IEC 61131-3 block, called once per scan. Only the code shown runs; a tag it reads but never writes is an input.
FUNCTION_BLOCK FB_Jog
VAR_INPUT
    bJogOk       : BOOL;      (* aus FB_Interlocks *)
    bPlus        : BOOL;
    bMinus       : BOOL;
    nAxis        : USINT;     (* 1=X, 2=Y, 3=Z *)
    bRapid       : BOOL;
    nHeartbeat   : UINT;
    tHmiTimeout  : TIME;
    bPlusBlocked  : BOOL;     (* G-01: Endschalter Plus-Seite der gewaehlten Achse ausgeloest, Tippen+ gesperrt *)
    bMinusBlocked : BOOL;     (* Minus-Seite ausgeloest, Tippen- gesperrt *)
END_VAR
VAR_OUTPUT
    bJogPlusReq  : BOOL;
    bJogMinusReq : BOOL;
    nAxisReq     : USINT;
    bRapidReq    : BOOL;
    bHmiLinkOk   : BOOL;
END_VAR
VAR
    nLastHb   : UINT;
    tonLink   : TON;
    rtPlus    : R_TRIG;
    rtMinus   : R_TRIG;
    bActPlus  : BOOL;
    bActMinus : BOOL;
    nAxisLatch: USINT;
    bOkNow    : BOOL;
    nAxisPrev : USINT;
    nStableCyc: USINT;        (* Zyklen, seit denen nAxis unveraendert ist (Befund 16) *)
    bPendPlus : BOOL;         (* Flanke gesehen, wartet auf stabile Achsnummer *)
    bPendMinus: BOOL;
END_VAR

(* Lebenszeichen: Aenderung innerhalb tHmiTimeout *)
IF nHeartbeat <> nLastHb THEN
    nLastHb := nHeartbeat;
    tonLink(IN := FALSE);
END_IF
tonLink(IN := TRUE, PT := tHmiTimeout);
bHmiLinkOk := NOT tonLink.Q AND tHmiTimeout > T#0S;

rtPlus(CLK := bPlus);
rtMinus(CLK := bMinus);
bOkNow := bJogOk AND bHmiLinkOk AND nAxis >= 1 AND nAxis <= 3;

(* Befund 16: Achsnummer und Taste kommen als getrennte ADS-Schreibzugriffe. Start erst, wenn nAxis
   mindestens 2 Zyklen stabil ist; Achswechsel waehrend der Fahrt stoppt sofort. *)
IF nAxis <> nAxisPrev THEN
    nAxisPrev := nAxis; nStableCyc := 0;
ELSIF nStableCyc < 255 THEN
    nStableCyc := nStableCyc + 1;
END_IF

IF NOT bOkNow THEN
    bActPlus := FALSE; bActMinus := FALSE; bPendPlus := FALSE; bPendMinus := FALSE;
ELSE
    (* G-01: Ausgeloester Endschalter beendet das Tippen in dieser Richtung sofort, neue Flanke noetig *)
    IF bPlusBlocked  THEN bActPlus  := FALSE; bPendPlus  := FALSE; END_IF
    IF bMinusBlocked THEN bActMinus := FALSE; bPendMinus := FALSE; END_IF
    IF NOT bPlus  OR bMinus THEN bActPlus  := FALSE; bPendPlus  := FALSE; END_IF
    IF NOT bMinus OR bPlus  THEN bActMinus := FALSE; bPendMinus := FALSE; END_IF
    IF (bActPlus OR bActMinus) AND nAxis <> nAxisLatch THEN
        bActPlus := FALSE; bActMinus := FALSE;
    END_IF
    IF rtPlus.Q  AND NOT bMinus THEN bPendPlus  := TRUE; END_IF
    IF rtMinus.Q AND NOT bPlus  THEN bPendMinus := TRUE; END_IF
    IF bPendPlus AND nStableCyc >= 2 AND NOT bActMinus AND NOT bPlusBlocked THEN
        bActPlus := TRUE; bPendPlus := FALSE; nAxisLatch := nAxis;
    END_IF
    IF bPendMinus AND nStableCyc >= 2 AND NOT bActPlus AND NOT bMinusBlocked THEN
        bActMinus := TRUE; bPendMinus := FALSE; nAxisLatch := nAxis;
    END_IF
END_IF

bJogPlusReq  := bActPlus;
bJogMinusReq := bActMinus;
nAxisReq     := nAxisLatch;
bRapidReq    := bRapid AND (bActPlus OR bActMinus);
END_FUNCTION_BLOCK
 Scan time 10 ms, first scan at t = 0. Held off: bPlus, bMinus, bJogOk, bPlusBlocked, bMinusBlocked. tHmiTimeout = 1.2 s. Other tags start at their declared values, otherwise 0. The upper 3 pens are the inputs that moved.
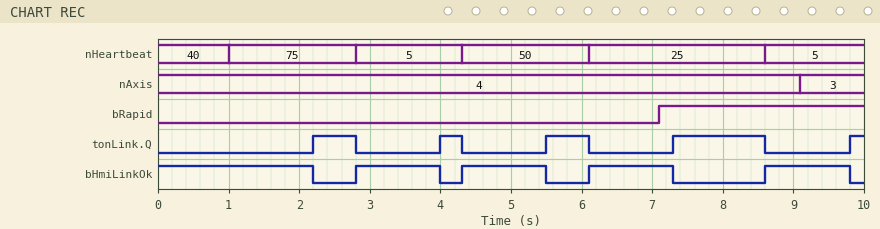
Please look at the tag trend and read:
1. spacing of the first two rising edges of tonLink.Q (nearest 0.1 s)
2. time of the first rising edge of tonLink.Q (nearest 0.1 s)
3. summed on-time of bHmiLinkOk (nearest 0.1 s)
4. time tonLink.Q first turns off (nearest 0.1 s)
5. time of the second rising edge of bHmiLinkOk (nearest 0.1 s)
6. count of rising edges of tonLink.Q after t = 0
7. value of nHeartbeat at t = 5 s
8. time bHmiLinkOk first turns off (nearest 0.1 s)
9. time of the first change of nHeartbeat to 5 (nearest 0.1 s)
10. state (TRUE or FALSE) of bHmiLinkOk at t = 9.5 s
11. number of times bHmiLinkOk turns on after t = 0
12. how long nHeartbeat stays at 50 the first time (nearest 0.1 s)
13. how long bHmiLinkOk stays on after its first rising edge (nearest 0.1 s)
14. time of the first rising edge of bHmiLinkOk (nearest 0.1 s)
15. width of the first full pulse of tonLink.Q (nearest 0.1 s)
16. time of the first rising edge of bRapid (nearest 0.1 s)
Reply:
1.8 s
2.2 s
7.0 s
2.8 s
4.3 s
5
50
2.2 s
2.8 s
TRUE
4
1.8 s
1.2 s
2.8 s
0.6 s
7.1 s
